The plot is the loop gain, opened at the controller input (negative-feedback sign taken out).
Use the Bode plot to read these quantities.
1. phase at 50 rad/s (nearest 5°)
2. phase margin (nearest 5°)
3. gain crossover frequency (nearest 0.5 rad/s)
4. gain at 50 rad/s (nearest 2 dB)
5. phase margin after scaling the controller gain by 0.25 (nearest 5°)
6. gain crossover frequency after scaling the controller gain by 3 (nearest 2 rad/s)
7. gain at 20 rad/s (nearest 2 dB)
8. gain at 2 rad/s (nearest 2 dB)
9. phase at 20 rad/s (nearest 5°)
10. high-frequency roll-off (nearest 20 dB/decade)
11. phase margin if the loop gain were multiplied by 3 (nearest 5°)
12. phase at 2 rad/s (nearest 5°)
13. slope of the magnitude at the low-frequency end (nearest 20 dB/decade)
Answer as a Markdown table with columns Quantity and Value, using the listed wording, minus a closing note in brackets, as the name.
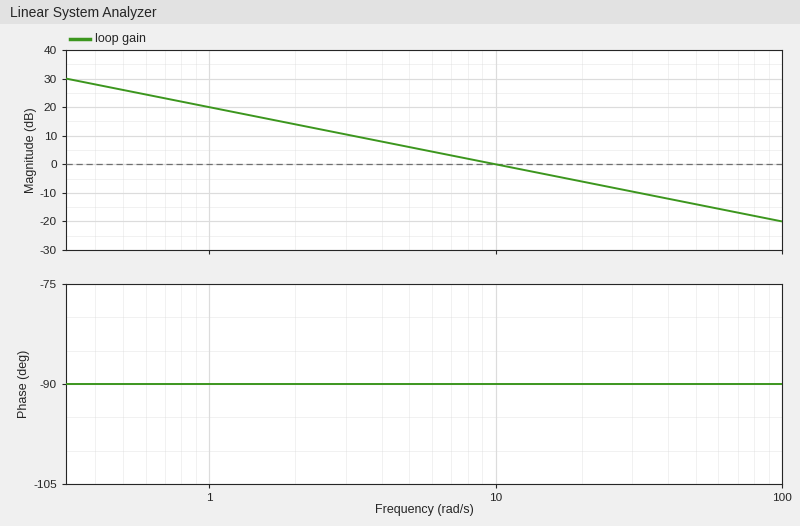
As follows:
| Quantity | Value |
|---|---|
| phase at 50 rad/s | -90° |
| phase margin | 90° |
| gain crossover frequency | 10.0 rad/s |
| gain at 50 rad/s | -14 dB |
| phase margin after scaling the controller gain by 0.25 | 90° |
| gain crossover frequency after scaling the controller gain by 3 | 30 rad/s |
| gain at 20 rad/s | -6 dB |
| gain at 2 rad/s | 14 dB |
| phase at 20 rad/s | -90° |
| high-frequency roll-off | -20 dB/decade |
| phase margin if the loop gain were multiplied by 3 | 90° |
| phase at 2 rad/s | -90° |
| slope of the magnitude at the low-frequency end | -20 dB/decade |
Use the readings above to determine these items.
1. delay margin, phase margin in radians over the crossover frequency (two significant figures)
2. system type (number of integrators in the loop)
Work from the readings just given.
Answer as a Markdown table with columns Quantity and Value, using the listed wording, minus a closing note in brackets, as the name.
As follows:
| Quantity | Value |
|---|---|
| delay margin, phase margin in radians over the crossover frequency | 0.16 s |
| system type | 1 |
